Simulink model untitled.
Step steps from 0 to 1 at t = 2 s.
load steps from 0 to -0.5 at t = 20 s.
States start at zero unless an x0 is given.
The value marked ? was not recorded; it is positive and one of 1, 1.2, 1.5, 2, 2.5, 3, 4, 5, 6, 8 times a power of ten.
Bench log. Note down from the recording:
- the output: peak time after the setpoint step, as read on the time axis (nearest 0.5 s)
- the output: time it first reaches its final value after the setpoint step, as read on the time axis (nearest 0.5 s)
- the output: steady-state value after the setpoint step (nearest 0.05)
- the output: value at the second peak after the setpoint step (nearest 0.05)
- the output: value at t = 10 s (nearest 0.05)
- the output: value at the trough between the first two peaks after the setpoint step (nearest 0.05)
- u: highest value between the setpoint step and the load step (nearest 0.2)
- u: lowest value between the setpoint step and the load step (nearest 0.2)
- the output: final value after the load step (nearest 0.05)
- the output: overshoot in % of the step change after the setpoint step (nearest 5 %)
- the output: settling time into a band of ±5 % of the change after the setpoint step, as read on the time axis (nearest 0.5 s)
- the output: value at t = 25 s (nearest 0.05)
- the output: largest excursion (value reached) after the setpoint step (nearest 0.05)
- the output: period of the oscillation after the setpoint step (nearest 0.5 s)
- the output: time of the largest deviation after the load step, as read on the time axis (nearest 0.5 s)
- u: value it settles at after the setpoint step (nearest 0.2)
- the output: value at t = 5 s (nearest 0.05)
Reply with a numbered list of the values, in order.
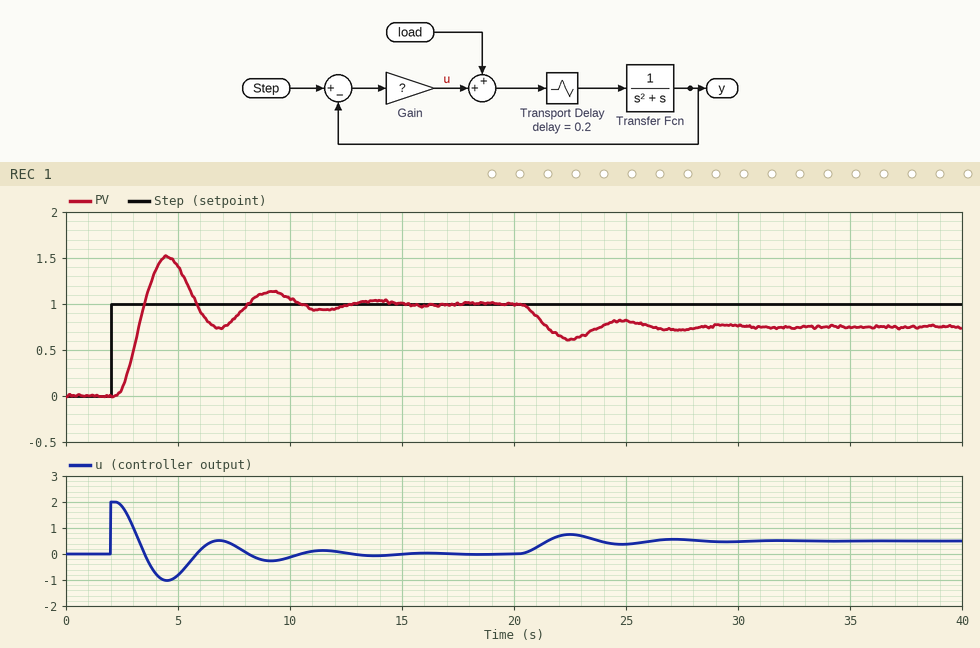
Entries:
1. 4.5 s
2. 3.5 s
3. 1.00
4. 1.15
5. 1.05
6. 0.75
7. 2.0
8. -1.0
9. 0.75
10. 50 %
11. 12.0 s
12. 0.80
13. 1.50
14. 4.5 s
15. 22.5 s
16. 0.0
17. 1.40
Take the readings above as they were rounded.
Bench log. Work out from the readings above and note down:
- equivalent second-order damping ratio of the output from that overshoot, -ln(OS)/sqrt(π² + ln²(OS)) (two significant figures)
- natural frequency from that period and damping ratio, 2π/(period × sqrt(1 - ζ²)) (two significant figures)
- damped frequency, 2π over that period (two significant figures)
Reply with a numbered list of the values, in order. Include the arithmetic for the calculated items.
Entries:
1. ln(0.5) = -0.693; 0.693 / sqrt(9.870 + 0.480) = 0.22
2. 2π / (4.5 × sqrt(1 - 0.22²)) = 1.4 rad/s
3. 2π / 4.5 = 1.4 rad/s
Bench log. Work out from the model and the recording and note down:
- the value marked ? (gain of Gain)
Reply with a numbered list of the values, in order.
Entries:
1. 2
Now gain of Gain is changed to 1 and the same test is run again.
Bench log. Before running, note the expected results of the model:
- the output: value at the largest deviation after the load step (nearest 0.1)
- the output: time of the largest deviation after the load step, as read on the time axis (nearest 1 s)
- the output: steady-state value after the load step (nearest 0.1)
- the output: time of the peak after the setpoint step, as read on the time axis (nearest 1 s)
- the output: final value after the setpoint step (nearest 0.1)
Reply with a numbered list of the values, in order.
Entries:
1. 0.4
2. 24 s
3. 0.5
4. 6 s
5. 1.0
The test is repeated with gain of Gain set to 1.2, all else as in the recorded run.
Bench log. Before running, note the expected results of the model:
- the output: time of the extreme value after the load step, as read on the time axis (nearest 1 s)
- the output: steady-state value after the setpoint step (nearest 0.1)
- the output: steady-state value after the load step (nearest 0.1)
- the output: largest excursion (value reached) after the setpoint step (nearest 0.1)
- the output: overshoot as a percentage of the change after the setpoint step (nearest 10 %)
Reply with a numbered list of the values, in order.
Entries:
1. 23 s
2. 1.0
3. 0.6
4. 1.3
5. 30 %
